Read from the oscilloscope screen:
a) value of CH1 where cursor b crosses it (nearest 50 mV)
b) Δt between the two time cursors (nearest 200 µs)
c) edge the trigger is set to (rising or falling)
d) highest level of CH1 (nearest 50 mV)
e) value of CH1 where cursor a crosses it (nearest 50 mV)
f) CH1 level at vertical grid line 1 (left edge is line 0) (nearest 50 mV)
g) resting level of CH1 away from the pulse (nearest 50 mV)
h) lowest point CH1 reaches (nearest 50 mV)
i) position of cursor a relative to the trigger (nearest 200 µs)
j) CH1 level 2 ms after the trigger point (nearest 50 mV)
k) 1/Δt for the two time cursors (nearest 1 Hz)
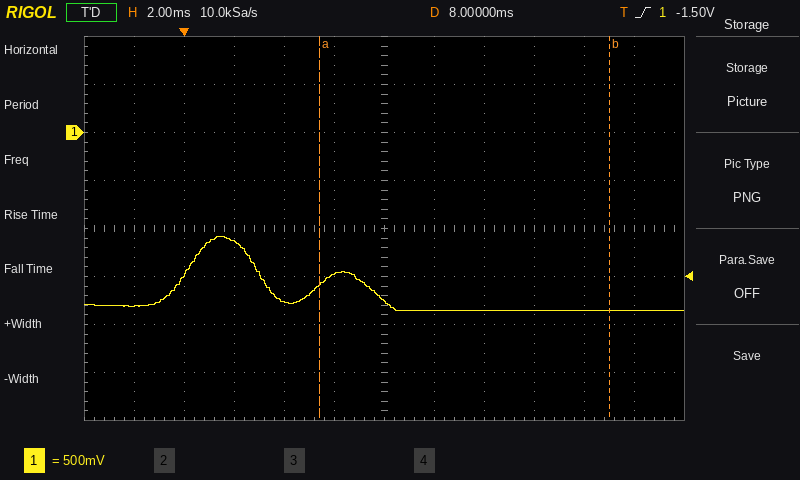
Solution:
-1.85 V
11.6 ms
rising
-1.10 V
-1.60 V
-1.80 V
-1.85 V
-1.85 V
+5.4 ms
-1.15 V
86 Hz
